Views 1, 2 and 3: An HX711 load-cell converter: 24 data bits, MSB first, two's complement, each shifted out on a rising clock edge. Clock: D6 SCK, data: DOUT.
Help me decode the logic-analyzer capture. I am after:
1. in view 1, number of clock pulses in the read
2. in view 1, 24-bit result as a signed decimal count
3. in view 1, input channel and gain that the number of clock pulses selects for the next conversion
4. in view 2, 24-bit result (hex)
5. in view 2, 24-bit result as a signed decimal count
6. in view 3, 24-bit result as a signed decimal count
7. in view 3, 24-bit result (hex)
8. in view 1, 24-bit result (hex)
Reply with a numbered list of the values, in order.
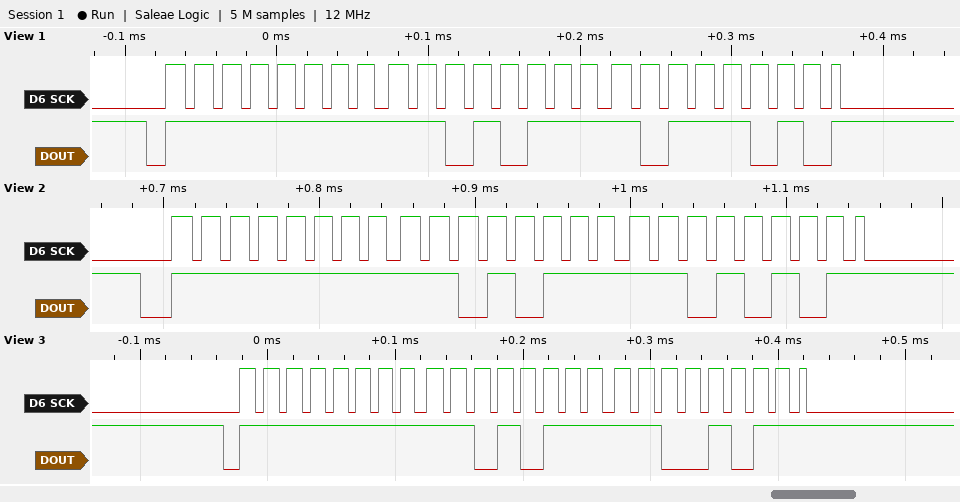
1. 25
2. -10310
3. channel A, gain 128
4. 0xFFD7D5
5. -10283
6. -10293
7. 0xFFD7CB
8. 0xFFD7BA
